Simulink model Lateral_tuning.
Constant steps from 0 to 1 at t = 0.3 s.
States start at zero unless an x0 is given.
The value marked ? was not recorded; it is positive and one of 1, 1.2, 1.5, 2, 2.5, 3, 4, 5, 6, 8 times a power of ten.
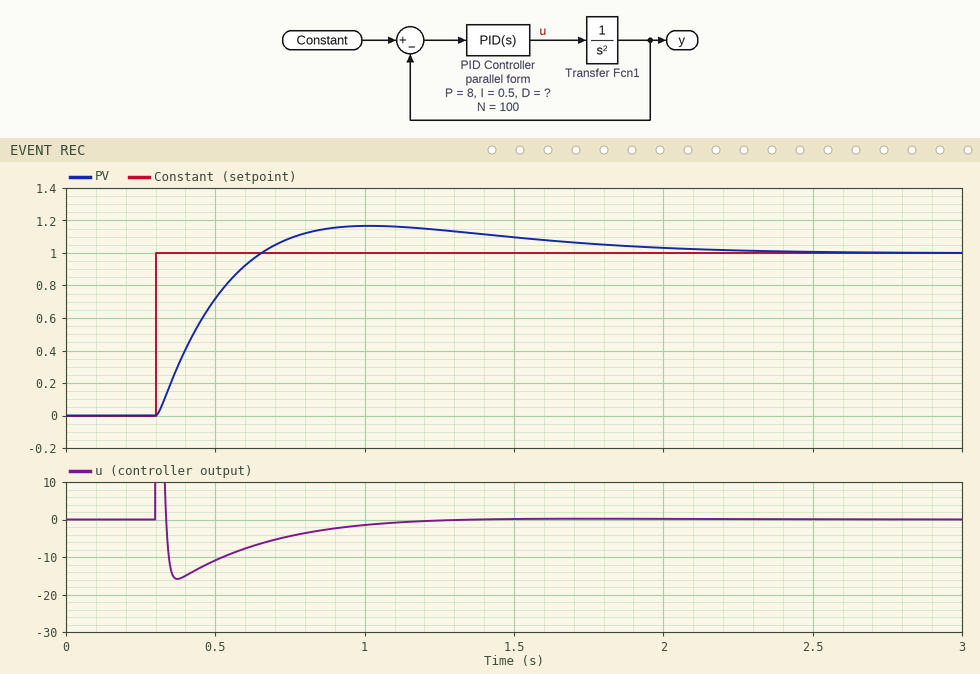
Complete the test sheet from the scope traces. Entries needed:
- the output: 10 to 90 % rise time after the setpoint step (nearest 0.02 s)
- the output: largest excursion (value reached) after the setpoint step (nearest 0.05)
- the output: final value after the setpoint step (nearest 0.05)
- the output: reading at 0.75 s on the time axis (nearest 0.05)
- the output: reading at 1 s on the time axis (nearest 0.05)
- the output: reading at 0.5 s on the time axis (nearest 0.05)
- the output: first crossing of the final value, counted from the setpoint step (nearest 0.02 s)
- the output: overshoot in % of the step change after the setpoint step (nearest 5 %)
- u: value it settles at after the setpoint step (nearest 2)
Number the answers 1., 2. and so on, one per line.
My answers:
1. 0.26 s
2. 1.15
3. 1.00
4. 1.10
5. 1.15
6. 0.70
7. 0.36 s
8. 15 %
9. 0
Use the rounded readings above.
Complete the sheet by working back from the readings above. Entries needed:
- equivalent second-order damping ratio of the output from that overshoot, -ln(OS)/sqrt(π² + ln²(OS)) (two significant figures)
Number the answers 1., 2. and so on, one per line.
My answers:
1. 0.52
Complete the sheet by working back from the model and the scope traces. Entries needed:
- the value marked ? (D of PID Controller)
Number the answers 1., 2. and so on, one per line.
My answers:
1. 5
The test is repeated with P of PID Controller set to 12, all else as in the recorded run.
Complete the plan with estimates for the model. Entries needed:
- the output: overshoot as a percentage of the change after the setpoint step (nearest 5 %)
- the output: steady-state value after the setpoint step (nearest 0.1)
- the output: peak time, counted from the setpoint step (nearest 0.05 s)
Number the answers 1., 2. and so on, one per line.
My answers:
1. 20 %
2. 1.0
3. 0.60 s
